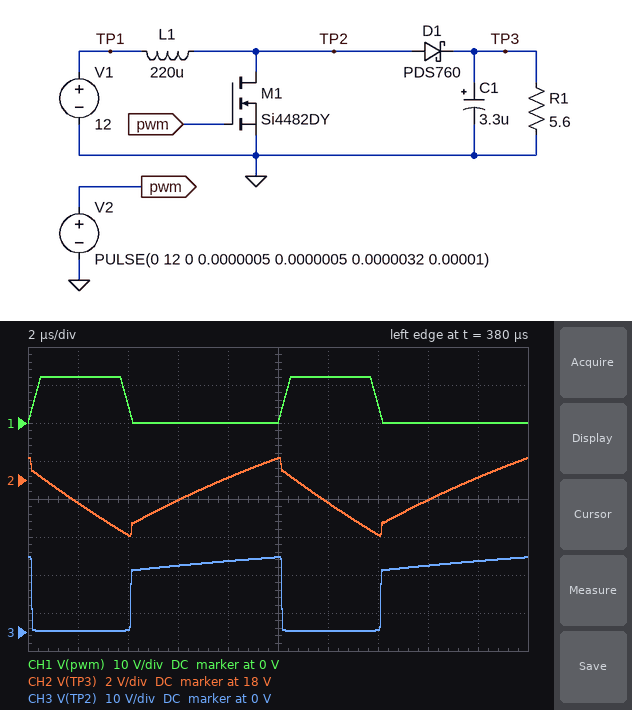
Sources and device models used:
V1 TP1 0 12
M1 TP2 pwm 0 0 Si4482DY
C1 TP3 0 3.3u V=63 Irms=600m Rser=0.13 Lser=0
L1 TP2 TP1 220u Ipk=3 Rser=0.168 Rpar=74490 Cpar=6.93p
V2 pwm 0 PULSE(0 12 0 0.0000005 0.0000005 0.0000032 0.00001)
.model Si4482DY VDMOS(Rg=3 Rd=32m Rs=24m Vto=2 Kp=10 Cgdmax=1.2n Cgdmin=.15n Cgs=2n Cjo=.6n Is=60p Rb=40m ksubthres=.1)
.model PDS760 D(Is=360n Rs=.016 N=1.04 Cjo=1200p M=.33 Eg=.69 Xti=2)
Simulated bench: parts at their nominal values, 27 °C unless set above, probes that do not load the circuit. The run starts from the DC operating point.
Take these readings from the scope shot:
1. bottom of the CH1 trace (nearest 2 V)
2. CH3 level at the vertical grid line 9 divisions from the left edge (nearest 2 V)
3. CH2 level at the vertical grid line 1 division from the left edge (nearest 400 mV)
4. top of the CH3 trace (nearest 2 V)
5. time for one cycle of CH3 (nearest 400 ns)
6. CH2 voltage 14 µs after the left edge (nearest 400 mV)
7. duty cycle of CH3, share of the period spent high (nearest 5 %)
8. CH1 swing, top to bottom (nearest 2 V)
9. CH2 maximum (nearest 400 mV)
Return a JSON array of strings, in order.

["0 V", "18 V", "16.8 V", "20 V", "10.0 µs", "15.2 V", "60 %", "12 V", "19.2 V"]
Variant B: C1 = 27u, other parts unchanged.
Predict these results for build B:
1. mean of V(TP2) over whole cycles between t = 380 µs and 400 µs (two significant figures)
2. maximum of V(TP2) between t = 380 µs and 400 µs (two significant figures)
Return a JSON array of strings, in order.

["12 V", "19 V"]
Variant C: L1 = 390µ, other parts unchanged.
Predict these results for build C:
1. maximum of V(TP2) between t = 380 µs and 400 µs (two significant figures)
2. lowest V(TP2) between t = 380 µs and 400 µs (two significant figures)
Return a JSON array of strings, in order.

["19 V", "320 mV"]
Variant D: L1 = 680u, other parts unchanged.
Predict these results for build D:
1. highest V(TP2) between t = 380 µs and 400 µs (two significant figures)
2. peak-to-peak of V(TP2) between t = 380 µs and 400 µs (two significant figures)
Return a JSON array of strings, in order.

["17 V", "16 V"]
